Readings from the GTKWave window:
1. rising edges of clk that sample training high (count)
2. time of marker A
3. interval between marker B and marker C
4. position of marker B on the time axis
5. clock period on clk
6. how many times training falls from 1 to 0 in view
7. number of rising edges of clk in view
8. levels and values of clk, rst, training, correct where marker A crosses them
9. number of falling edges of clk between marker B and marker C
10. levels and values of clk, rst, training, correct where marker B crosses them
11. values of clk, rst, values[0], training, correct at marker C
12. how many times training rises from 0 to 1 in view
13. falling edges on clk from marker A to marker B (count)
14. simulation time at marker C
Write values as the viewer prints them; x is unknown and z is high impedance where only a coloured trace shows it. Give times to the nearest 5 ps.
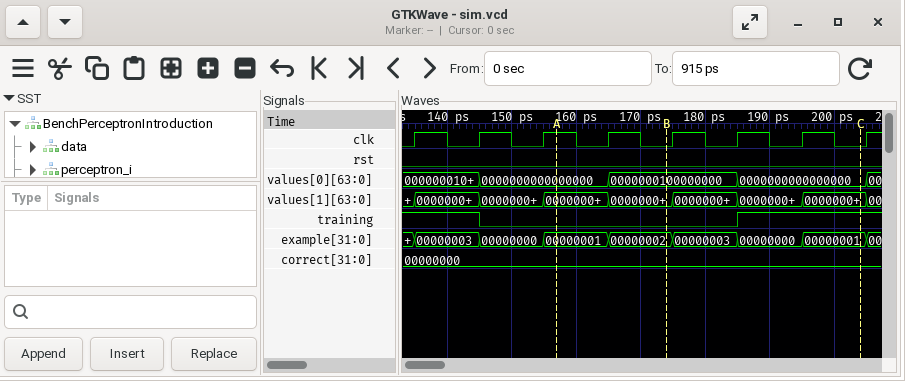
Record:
4
155 ps
30 ps
175 ps
10 ps
1
8
clk=1, rst=0, training=0, correct=00000000
3
clk=0, rst=0, training=0, correct=00000000
clk=0, rst=0, values[0]=0000000000000000, training=1, correct=00000000
1
2
205 ps
